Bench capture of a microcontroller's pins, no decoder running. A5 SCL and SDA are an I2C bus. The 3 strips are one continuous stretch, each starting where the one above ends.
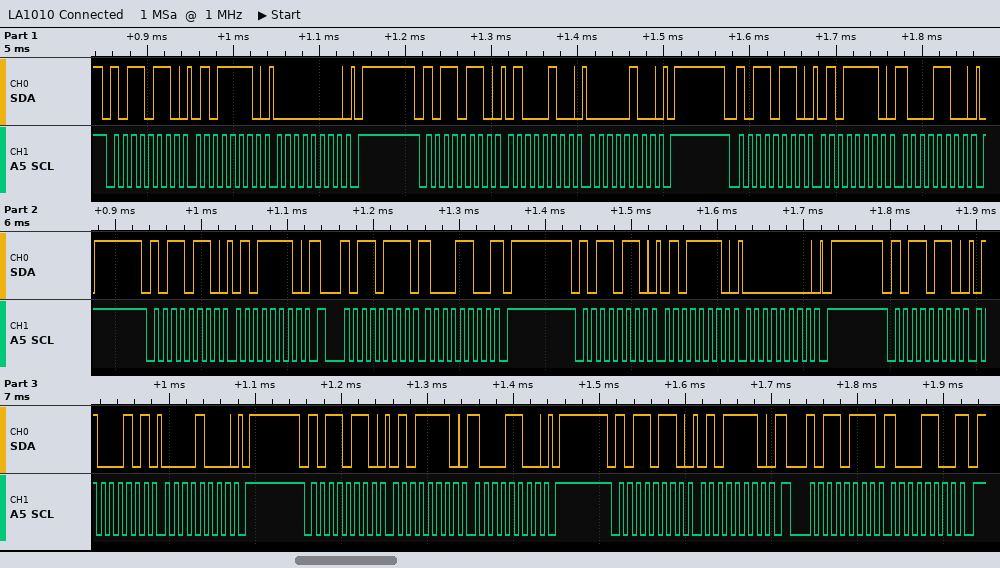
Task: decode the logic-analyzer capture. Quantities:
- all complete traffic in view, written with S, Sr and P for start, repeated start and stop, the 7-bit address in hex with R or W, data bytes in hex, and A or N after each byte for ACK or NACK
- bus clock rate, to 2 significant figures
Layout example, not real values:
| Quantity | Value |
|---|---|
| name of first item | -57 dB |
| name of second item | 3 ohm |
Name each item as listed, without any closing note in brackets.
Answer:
| Quantity | Value |
|---|---|
| all complete traffic in view, written with S, Sr and P for start, repeated start and stop, the 7-bit address in hex with R or W, data bytes in hex, and A or N after each byte for ACK or NACK | S 5BW A 5E A 00 A P S 5BW A 44 A 04 A P S 5BW A 5E A 8C A P S 5BW A 5E A Sr 5BR A 8C N P S 5BW A 5E A 00 A P S 5BW A 45 A 08 A P S 5BW A 5E A 8C A P S 5BW A 5E A Sr 5BR A 8C N P |
| bus clock rate, to 2 significant figures | 100 kHz |
